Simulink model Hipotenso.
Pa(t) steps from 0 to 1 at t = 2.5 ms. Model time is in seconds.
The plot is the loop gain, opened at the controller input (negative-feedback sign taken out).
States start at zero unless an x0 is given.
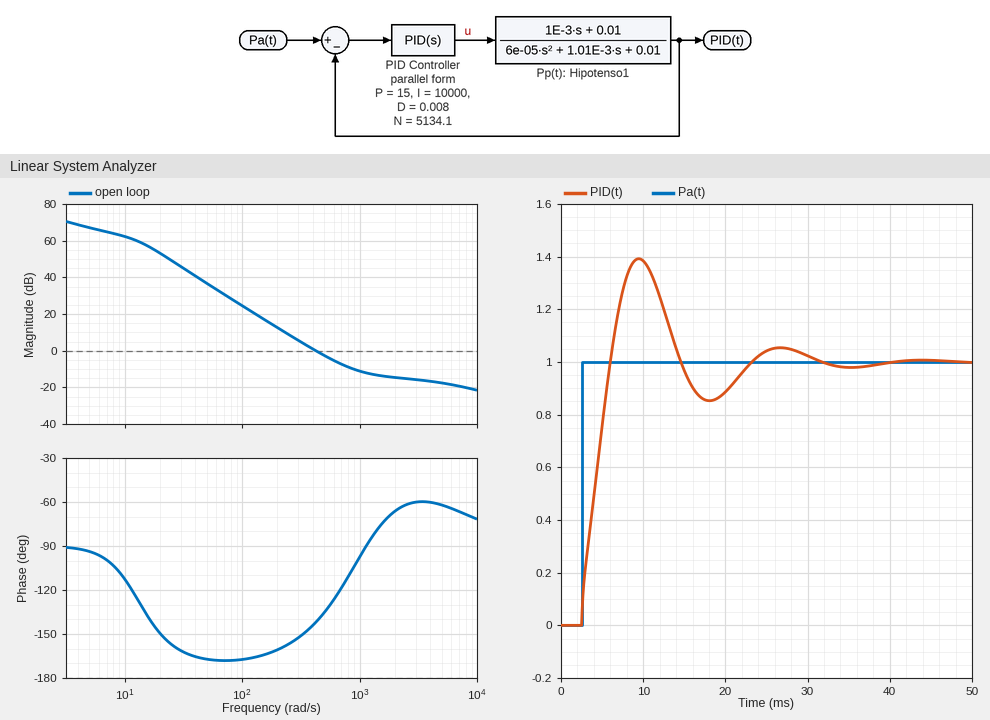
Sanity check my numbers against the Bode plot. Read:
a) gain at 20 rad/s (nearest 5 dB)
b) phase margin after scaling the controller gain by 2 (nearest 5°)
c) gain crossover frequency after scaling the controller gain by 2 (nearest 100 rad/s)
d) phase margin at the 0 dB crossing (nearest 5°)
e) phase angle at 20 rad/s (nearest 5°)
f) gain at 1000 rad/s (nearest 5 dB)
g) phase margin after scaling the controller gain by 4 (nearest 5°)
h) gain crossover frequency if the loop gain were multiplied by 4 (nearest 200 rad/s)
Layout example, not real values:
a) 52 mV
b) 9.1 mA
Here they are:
a) 55 dB
b) 55°
c) 600 rad/s
d) 40°
e) -150°
f) -10 dB
g) 90°
h) 1200 rad/s
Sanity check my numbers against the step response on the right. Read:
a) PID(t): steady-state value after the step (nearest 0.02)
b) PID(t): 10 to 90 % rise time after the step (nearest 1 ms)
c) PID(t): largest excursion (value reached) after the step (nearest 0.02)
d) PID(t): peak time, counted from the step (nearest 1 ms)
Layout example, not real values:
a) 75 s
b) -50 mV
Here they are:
a) 1.00
b) 3 ms
c) 1.40
d) 7 ms
